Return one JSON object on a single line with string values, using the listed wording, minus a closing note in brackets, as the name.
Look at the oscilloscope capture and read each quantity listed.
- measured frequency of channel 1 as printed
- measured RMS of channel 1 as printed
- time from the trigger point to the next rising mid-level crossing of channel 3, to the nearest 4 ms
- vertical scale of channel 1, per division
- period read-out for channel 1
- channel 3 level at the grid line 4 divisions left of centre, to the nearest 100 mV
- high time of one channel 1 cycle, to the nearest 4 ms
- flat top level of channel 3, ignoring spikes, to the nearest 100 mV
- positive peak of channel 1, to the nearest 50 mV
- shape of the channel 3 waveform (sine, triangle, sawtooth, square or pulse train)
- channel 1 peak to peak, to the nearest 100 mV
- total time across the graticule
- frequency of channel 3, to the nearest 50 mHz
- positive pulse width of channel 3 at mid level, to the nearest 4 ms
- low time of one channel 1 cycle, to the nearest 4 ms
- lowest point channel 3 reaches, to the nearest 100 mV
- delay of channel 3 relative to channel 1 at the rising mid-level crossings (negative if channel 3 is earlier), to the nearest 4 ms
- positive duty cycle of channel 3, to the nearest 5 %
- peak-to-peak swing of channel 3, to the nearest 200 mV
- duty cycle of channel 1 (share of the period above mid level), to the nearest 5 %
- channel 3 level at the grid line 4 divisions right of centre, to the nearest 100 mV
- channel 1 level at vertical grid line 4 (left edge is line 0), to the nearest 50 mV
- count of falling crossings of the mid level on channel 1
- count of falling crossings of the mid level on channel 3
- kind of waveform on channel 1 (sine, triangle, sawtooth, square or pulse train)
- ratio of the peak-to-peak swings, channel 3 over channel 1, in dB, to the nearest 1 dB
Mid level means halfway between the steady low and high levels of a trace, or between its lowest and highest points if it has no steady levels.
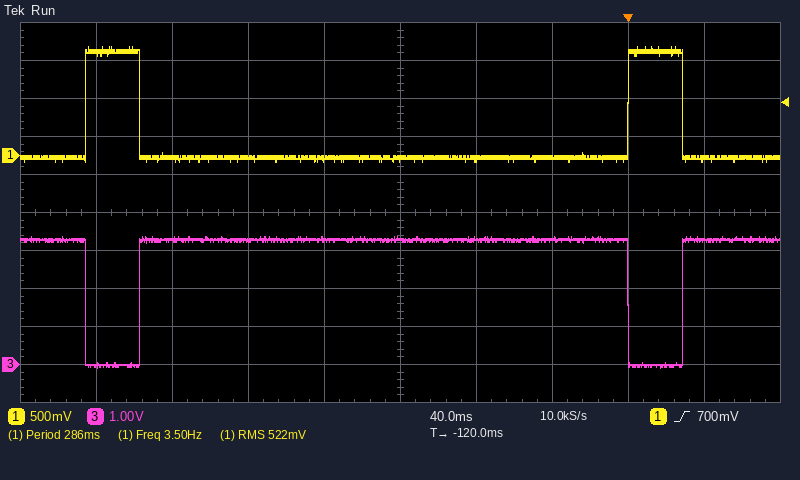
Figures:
{"measured frequency of channel 1 as printed": "3.50 Hz", "measured RMS of channel 1 as printed": "522 mV", "time from the trigger point to the next rising mid-level crossing of channel 3, to the nearest 4 ms": "28 ms", "vertical scale of channel 1, per division": "500 mV", "period read-out for channel 1": "286 ms", "channel 3 level at the grid line 4 divisions left of centre, to the nearest 100 mV": "0.0 V", "high time of one channel 1 cycle, to the nearest 4 ms": "28 ms", "flat top level of channel 3, ignoring spikes, to the nearest 100 mV": "3.3 V", "positive peak of channel 1, to the nearest 50 mV": "1.45 V", "shape of the channel 3 waveform": "pulse train", "channel 1 peak to peak, to the nearest 100 mV": "1.50 V", "total time across the graticule": "400 ms", "frequency of channel 3, to the nearest 50 mHz": "3.50 Hz", "positive pulse width of channel 3 at mid level, to the nearest 4 ms": "256 ms", "low time of one channel 1 cycle, to the nearest 4 ms": "256 ms", "lowest point channel 3 reaches, to the nearest 100 mV": "-100 mV", "delay of channel 3 relative to channel 1 at the rising mid-level crossings (negative if channel 3 is earlier), to the nearest 4 ms": "+28 ms", "positive duty cycle of channel 3, to the nearest 5 %": "90 %", "peak-to-peak swing of channel 3, to the nearest 200 mV": "3.4 V", "duty cycle of channel 1 (share of the period above mid level), to the nearest 5 %": "10 %", "channel 3 level at the grid line 4 divisions right of centre, to the nearest 100 mV": "3.3 V", "channel 1 level at vertical grid line 4 (left edge is line 0), to the nearest 50 mV": "-50 mV", "count of falling crossings of the mid level on channel 1": "2", "count of falling crossings of the mid level on channel 3": "2", "kind of waveform on channel 1": "pulse train", "ratio of the peak-to-peak swings, channel 3 over channel 1, in dB, to the nearest 1 dB": "7 dB"}
